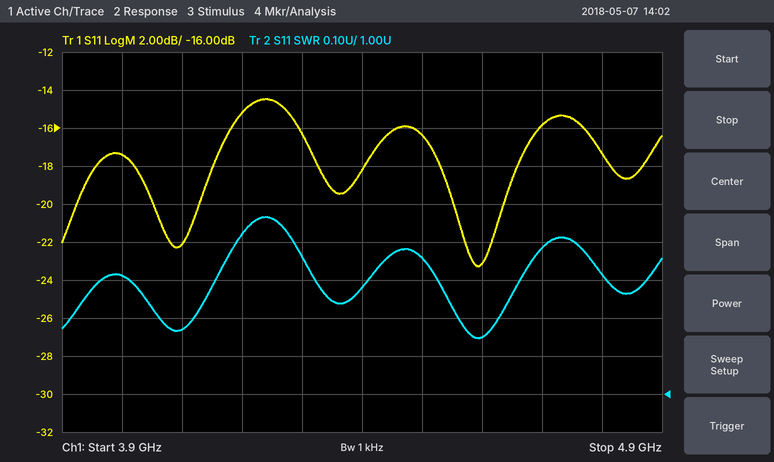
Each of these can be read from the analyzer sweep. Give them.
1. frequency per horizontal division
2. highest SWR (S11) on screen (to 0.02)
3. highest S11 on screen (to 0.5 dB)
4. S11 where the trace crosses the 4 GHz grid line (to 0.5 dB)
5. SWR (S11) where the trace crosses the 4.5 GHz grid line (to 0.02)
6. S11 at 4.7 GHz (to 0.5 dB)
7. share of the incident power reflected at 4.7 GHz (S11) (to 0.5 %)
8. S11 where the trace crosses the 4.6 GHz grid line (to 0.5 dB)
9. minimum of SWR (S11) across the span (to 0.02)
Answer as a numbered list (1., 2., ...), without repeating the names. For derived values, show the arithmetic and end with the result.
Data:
1. 100 MHz
2. 1.46
3. -14.5 dB
4. -17.5 dB
5. 1.36
6. -16.0 dB
7. 10^(-16/10) ≈ 2.5 %
8. -23.0 dB
9. 1.14
